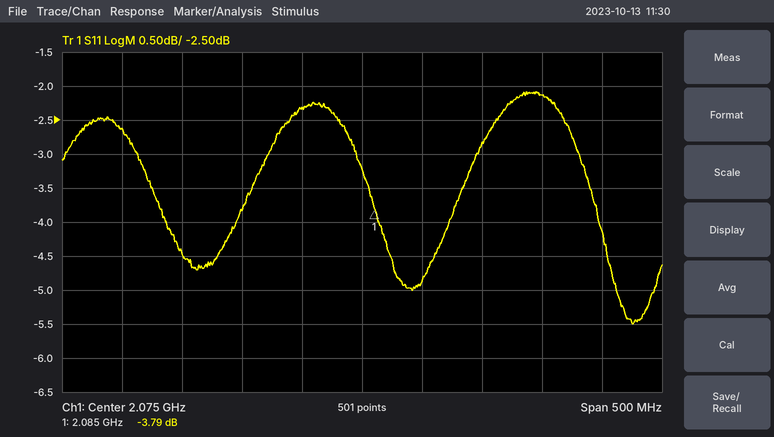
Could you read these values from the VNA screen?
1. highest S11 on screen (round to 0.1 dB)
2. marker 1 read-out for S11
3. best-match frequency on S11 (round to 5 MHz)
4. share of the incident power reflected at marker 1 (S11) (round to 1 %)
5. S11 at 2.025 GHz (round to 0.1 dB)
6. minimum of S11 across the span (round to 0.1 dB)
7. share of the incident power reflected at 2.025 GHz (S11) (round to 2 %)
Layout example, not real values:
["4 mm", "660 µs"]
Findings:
["-2.1 dB", "-3.79 dB", "2.300 GHz", "42 %", "-2.3 dB", "-5.5 dB", "58 %"]
